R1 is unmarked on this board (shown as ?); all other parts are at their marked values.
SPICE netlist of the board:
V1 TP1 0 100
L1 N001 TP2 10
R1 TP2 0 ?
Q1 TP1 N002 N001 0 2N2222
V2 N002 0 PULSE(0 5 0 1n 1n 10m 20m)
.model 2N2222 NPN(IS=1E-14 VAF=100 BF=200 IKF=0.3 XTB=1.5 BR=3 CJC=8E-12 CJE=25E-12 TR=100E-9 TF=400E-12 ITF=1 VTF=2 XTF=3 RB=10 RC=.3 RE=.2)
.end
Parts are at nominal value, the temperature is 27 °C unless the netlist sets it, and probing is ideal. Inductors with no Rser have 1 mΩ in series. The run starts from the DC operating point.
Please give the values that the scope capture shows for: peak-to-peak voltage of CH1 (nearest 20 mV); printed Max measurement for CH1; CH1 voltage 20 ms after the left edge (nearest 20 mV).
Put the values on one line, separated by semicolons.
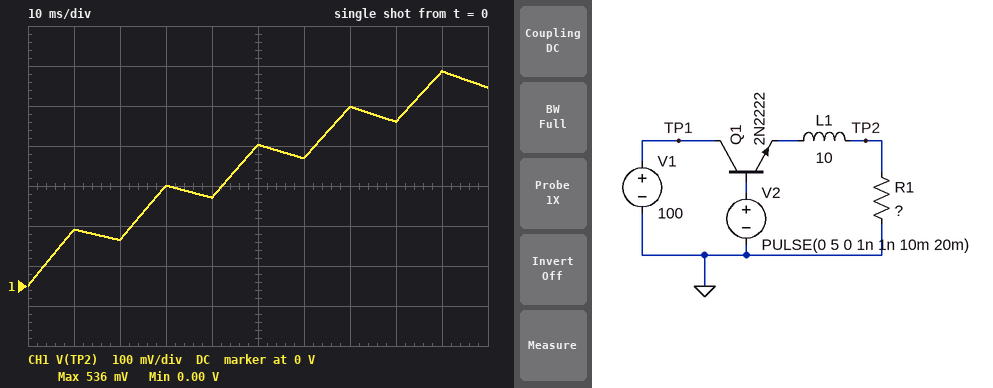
540 mV; 536 mV; 120 mV
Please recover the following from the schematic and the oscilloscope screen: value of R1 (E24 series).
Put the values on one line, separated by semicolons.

33 Ω
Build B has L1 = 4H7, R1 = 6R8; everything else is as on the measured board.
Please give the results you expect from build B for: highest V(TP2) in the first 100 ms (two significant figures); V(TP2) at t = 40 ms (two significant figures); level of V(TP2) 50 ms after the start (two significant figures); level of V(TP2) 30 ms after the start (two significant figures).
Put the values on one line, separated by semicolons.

250 mV; 100 mV; 160 mV; 110 mV
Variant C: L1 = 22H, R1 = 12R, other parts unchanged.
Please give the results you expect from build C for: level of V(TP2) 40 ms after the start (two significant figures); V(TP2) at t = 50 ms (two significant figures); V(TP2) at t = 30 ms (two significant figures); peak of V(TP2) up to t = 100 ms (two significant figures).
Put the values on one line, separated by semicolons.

40 mV; 63 mV; 44 mV; 100 mV
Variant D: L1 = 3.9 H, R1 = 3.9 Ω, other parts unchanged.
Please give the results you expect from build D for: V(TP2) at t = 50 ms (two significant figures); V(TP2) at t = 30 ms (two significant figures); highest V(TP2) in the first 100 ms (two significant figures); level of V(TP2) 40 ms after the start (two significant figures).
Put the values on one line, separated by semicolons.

110 mV; 78 mV; 180 mV; 70 mV
